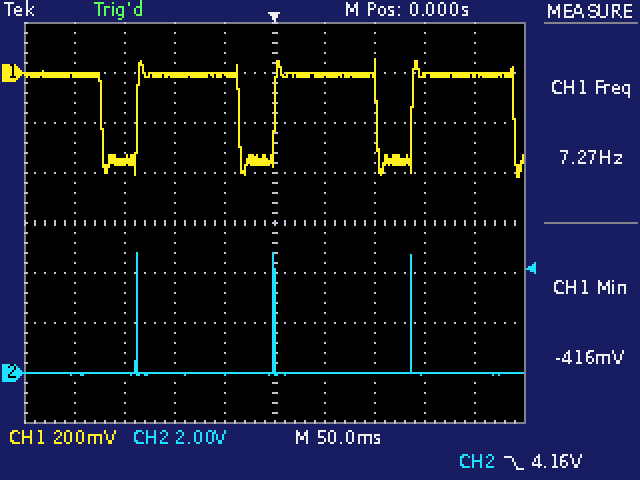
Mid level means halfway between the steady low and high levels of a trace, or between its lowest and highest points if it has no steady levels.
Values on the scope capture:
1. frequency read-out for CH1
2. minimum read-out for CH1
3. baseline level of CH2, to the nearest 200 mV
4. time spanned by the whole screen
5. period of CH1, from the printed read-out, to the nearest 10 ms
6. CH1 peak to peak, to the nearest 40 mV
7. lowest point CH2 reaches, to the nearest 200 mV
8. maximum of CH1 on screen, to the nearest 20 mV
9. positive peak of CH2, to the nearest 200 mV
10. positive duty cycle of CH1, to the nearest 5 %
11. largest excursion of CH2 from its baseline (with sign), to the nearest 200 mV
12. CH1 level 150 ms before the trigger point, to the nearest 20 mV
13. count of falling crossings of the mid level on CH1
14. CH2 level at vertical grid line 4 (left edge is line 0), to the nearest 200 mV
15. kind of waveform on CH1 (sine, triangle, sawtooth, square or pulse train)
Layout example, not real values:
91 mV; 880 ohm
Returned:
7.27 Hz; -416 mV; 0.0 V; 500 ms; 140 ms; 480 mV; 0.0 V; 60 mV; 4.8 V; 75 %; +4.8 V; -340 mV; 4; 0.0 V; pulse train
